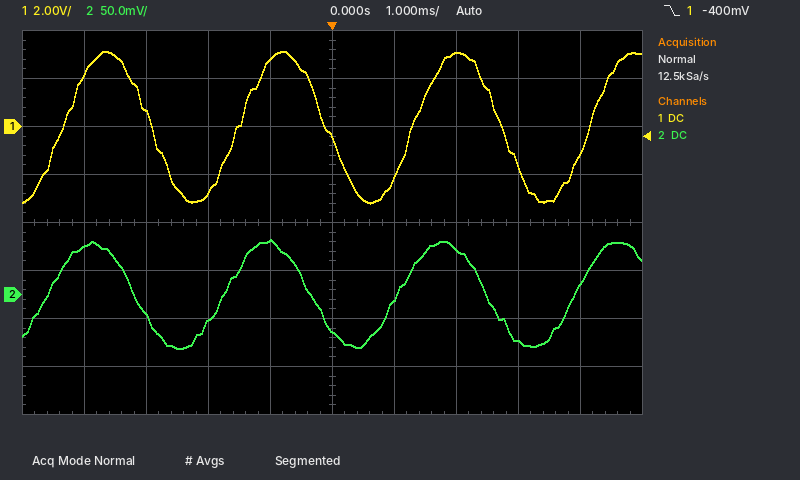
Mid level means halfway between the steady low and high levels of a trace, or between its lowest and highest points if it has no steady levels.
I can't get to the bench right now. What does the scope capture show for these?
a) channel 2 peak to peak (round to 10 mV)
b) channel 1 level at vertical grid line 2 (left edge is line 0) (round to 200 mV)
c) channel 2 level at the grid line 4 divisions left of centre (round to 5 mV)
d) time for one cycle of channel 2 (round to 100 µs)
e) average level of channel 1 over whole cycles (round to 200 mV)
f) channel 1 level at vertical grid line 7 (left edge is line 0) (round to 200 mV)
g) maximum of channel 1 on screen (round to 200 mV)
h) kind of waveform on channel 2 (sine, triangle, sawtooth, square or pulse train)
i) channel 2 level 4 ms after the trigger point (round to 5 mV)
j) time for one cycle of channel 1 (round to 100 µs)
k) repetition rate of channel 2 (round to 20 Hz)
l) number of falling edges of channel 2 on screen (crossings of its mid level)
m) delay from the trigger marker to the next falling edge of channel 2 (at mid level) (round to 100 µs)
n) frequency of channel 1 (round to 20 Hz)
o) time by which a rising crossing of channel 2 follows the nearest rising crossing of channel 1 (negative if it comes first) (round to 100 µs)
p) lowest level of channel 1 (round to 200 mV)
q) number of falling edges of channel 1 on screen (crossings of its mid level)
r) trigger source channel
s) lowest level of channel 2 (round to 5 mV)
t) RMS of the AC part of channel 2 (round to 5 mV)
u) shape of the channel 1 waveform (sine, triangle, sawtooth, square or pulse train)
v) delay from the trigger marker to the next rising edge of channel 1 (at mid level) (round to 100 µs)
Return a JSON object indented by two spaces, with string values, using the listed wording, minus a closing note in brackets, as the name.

{
  "channel 2 peak to peak": "110 mV",
  "channel 1 level at vertical grid line 2 (left edge is line 0)": "600 mV",
  "channel 2 level at the grid line 4 divisions left of centre": "50 mV",
  "time for one cycle of channel 2": "2.8 ms",
  "average level of channel 1 over whole cycles": "0.0 V",
  "channel 1 level at vertical grid line 7 (left edge is line 0)": "3.0 V",
  "maximum of channel 1 on screen": "3.2 V",
  "kind of waveform on channel 2": "sine",
  "channel 2 level 4 ms after the trigger point": "10 mV",
  "time for one cycle of channel 1": "2.8 ms",
  "repetition rate of channel 2": "360 Hz",
  "number of falling edges of channel 2 on screen": "3",
  "delay from the trigger marker to the next falling edge of channel 2 (at mid level)": "2.5 ms",
  "frequency of channel 1": "360 Hz",
  "time by which a rising crossing of channel 2 follows the nearest rising crossing of channel 1 (negative if it comes first)": "-200 µs",
  "lowest level of channel 1": "-3.2 V",
  "number of falling edges of channel 1 on screen": "3",
  "trigger source channel": "channel 1",
  "lowest level of channel 2": "-55 mV",
  "RMS of the AC part of channel 2": "40 mV",
  "shape of the channel 1 waveform": "sine",
  "delay from the trigger marker to the next rising edge of channel 1 (at mid level)": "1.3 ms"
}
